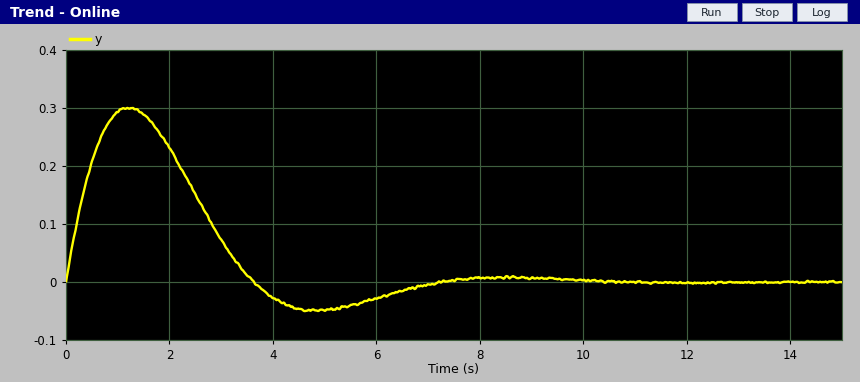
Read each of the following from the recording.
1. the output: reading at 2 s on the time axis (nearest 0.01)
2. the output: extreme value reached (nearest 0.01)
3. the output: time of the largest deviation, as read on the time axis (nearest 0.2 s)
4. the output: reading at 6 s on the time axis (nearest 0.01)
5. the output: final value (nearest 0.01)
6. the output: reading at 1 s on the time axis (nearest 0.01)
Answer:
0.23
0.30
1.2 s
-0.03
0.00
0.29
